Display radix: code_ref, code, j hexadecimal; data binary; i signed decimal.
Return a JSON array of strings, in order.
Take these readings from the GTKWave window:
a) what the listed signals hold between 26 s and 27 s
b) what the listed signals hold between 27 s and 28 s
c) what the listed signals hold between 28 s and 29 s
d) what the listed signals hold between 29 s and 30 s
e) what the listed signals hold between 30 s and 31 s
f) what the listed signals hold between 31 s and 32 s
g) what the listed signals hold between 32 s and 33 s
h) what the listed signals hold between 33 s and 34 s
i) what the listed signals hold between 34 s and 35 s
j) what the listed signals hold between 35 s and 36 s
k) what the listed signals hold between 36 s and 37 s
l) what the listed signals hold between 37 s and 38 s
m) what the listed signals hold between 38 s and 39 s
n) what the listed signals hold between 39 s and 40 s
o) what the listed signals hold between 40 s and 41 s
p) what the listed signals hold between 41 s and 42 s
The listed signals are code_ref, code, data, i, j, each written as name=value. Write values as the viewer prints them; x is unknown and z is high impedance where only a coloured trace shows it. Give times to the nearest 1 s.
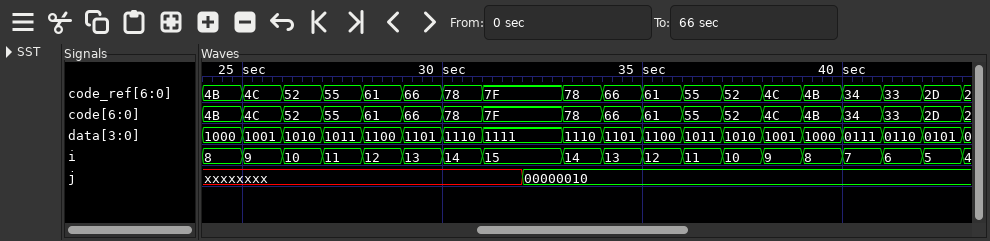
["code_ref=52, code=52, data=1010, i=10, j=xxxxxxxx", "code_ref=55, code=55, data=1011, i=11, j=xxxxxxxx", "code_ref=61, code=61, data=1100, i=12, j=xxxxxxxx", "code_ref=66, code=66, data=1101, i=13, j=xxxxxxxx", "code_ref=78, code=78, data=1110, i=14, j=xxxxxxxx", "code_ref=7F, code=7F, data=1111, i=15, j=xxxxxxxx", "code_ref=7F, code=7F, data=1111, i=15, j=00000010", "code_ref=78, code=78, data=1110, i=14, j=00000010", "code_ref=66, code=66, data=1101, i=13, j=00000010", "code_ref=61, code=61, data=1100, i=12, j=00000010", "code_ref=55, code=55, data=1011, i=11, j=00000010", "code_ref=52, code=52, data=1010, i=10, j=00000010", "code_ref=4C, code=4C, data=1001, i=9, j=00000010", "code_ref=4B, code=4B, data=1000, i=8, j=00000010", "code_ref=34, code=34, data=0111, i=7, j=00000010", "code_ref=33, code=33, data=0110, i=6, j=00000010"]
